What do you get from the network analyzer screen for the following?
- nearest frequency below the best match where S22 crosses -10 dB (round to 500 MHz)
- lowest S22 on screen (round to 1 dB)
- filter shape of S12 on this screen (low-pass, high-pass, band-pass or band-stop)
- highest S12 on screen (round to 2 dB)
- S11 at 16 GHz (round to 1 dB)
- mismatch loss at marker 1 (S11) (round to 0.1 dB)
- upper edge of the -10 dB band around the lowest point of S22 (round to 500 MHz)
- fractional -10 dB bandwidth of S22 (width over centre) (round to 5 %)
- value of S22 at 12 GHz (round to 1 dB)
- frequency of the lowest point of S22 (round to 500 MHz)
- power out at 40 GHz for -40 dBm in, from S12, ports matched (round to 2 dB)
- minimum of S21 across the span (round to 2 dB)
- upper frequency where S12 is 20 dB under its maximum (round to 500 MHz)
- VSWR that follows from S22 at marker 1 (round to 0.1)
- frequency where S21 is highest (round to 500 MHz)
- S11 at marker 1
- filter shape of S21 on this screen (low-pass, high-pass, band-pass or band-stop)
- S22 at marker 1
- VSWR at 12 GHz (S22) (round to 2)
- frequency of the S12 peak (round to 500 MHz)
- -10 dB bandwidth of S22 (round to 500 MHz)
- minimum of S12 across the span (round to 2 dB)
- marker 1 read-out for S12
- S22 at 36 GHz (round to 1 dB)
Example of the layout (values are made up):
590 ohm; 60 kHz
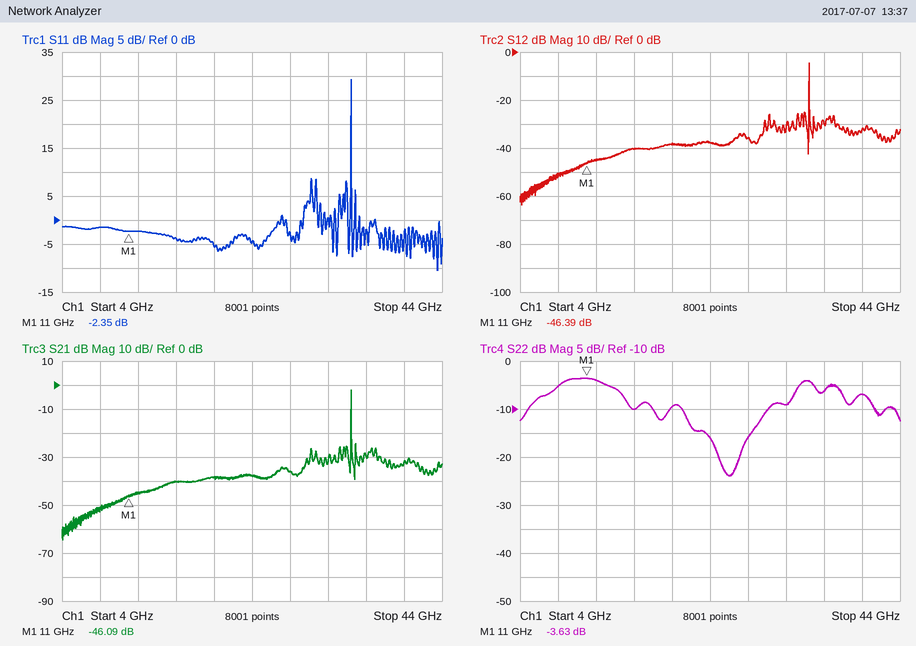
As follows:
21.0 GHz; -24 dB; band-pass; -4 dB; -4 dB; 3.8 dB; 30.0 GHz; 35 %; -4 dB; 26.0 GHz; -72 dBm; -64 dB; 34.5 GHz; 4.9; 34.5 GHz; -2.35 dB; band-pass; -3.63 dB; 4; 34.5 GHz; 9.0 GHz; -64 dB; -46.39 dB; -6 dB
